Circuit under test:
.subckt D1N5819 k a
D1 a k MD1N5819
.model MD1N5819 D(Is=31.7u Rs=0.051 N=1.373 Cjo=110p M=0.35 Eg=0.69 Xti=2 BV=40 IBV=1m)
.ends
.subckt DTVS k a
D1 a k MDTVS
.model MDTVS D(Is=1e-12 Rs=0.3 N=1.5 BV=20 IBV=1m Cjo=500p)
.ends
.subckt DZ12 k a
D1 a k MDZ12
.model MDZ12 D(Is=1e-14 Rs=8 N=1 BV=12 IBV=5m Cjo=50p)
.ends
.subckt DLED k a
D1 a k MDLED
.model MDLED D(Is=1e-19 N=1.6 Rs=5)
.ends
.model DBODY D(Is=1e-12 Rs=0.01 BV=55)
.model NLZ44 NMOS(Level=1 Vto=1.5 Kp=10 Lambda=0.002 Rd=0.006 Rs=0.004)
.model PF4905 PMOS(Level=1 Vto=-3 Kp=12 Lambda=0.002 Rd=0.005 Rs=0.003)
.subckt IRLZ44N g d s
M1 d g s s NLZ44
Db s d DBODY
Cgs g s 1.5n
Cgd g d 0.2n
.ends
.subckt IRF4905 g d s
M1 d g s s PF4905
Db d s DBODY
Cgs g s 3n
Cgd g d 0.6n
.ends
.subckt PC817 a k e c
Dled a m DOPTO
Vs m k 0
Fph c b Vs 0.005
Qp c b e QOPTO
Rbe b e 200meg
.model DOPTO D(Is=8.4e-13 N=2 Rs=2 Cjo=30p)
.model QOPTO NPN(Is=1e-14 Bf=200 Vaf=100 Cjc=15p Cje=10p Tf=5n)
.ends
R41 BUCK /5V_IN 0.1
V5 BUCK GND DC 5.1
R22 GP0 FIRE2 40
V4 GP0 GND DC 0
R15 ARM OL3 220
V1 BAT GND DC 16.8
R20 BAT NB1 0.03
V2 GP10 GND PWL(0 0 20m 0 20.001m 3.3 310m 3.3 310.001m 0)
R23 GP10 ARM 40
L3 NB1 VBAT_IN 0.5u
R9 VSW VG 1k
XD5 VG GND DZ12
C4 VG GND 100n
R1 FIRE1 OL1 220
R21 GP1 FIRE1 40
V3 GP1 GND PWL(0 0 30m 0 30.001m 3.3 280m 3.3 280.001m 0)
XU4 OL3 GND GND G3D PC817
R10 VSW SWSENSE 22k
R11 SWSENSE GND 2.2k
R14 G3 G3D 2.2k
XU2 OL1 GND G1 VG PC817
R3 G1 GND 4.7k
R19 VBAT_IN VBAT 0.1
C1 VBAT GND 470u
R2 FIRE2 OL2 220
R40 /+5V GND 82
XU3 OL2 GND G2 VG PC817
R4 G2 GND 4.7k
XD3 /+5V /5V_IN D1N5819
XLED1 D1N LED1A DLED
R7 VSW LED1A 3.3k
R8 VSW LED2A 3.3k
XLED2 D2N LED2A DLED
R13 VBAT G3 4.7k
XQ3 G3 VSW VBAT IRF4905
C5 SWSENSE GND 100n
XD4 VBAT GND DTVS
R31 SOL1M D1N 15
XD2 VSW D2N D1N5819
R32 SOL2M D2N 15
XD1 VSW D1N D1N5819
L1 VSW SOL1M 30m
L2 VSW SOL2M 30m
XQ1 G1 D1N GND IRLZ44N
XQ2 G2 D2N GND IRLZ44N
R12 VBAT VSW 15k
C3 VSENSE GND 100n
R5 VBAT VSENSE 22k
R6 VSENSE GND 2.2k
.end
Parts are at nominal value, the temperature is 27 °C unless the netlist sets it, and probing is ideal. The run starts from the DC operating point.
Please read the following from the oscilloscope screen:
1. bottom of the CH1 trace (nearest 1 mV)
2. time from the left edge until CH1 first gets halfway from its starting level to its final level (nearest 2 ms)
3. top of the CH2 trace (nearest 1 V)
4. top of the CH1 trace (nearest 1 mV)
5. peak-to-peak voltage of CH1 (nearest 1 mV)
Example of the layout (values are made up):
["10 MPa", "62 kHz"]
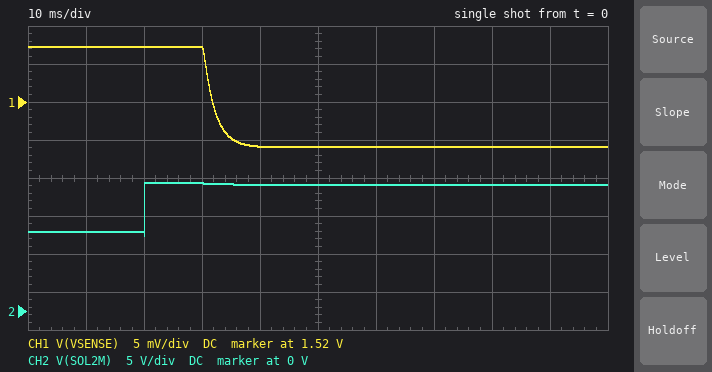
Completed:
["1.514 V", "32 ms", "17 V", "1.527 V", "13 mV"]
